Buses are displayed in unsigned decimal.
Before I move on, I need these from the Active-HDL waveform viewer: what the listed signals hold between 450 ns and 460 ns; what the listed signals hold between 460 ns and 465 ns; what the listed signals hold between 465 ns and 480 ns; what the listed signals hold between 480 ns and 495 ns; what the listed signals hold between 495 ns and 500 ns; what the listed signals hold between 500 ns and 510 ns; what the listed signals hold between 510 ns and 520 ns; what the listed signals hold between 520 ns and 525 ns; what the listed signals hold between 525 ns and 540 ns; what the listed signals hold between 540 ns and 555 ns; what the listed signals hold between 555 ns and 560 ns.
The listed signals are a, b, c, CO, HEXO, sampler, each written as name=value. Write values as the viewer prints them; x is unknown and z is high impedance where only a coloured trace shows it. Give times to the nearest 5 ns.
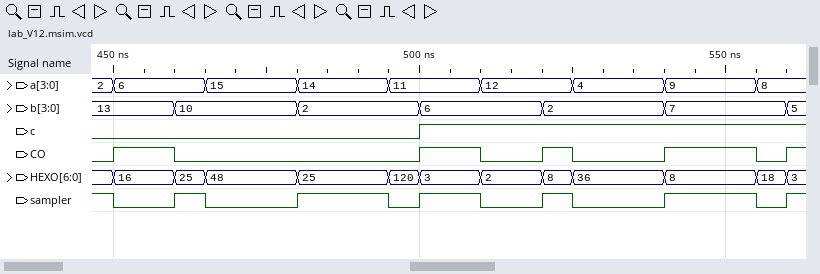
a=6, b=13, c=0, CO=1, HEXO=16, sampler=0
a=6, b=10, c=0, CO=0, HEXO=25, sampler=1
a=15, b=10, c=0, CO=0, HEXO=48, sampler=0
a=14, b=2, c=0, CO=0, HEXO=25, sampler=1
a=11, b=2, c=0, CO=0, HEXO=120, sampler=0
a=11, b=6, c=1, CO=1, HEXO=3, sampler=1
a=12, b=6, c=1, CO=0, HEXO=2, sampler=0
a=12, b=2, c=1, CO=1, HEXO=8, sampler=1
a=4, b=2, c=1, CO=0, HEXO=36, sampler=0
a=9, b=7, c=1, CO=1, HEXO=8, sampler=1
a=8, b=7, c=1, CO=0, HEXO=18, sampler=0
